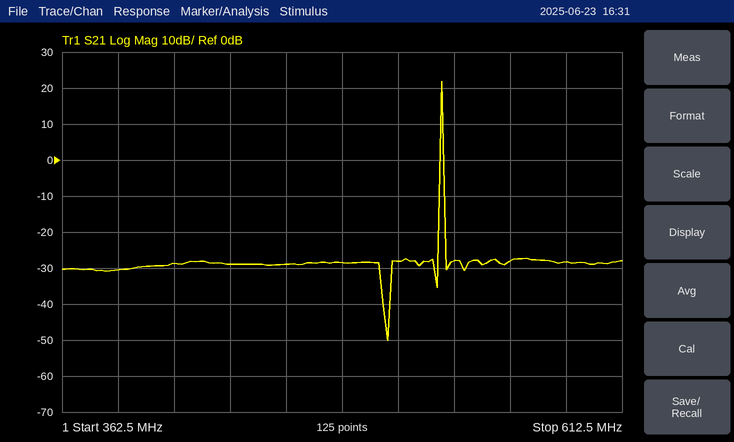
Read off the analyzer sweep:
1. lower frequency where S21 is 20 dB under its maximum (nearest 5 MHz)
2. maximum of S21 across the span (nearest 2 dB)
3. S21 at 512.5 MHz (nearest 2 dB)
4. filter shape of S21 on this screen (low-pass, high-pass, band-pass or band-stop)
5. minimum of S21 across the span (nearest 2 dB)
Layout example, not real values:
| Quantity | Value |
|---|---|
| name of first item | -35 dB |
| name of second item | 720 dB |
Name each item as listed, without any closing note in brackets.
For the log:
| Quantity | Value |
|---|---|
| lower frequency where S21 is 20 dB under its maximum | 530 MHz |
| maximum of S21 across the span | 22 dB |
| S21 at 512.5 MHz | -28 dB |
| filter shape of S21 on this screen | band-pass |
| minimum of S21 across the span | -50 dB |
